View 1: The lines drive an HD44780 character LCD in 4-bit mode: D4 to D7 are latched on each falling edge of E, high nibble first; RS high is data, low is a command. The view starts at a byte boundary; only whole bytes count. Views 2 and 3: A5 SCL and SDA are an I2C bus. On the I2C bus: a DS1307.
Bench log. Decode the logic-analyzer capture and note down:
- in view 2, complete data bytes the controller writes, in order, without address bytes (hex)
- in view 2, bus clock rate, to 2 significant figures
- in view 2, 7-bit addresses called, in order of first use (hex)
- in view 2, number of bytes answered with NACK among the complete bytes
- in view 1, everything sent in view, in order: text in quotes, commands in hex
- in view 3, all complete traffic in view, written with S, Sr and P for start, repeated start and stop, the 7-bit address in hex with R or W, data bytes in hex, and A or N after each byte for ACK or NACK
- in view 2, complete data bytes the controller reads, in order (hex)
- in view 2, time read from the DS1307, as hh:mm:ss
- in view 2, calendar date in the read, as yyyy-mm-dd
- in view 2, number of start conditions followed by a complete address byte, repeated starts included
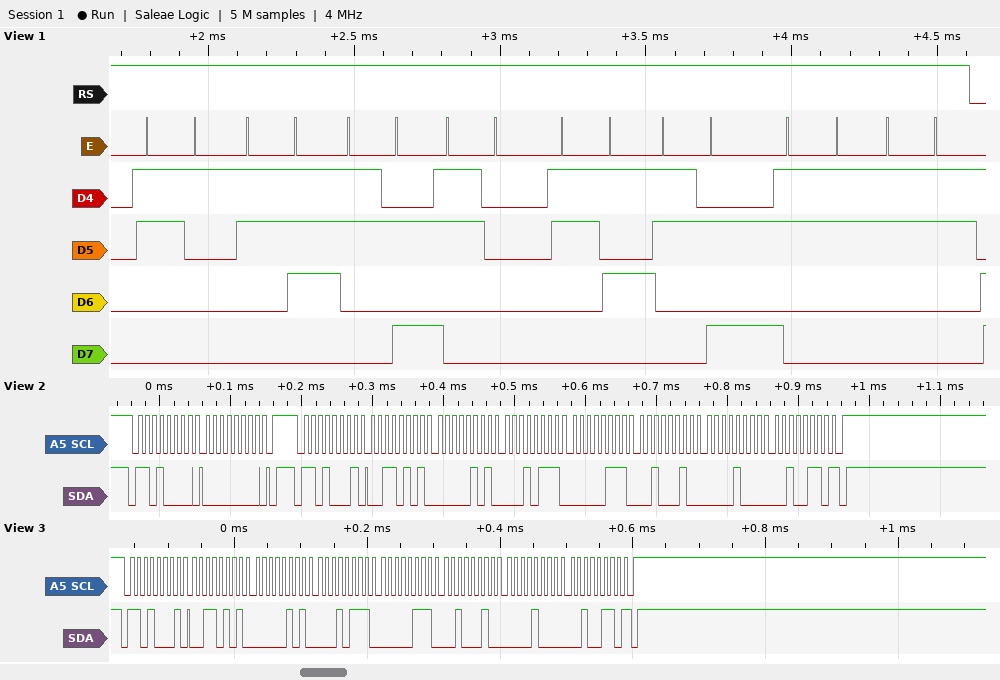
00
100 kHz
0x68
1
"17:05:33"
S 68R A 35 A 05 A 17 A 07 A 22 A 08 A 26 N P
35 05 17 07 22 08 26
17:05:35
2026-08-22
2
